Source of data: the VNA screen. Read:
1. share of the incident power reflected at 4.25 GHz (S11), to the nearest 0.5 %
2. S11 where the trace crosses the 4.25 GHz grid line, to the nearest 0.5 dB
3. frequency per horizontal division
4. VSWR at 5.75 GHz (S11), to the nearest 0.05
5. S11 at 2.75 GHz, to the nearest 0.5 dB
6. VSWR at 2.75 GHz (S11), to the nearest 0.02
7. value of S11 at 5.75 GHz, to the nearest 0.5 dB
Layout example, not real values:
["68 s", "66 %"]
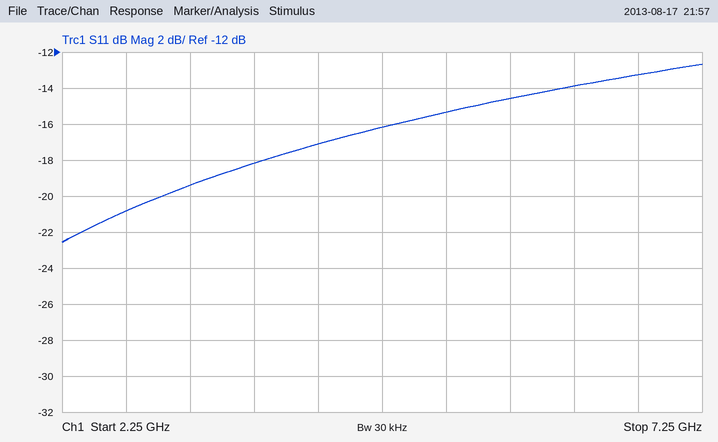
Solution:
["2.0 %", "-17.0 dB", "500 MHz", "1.45", "-21.0 dB", "1.20", "-14.5 dB"]
